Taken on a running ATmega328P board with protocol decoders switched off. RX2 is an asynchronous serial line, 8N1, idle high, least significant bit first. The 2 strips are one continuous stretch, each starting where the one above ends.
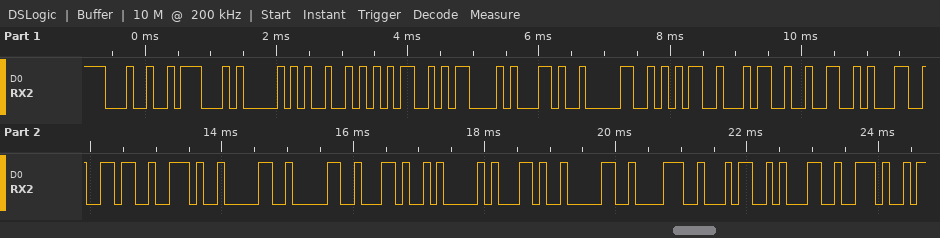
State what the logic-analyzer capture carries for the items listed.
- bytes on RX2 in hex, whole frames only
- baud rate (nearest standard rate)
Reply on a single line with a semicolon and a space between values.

0x24 0x47 0x50 0x52 0x4D 0x43 0x2C 0x30 0x35 0x34 0x32 0x31 0x36 0x2E 0x30 0x30 0x2C 0x41 0x2C 0x30 0x38 0x34 0x31 0x2E; 9600 baud
